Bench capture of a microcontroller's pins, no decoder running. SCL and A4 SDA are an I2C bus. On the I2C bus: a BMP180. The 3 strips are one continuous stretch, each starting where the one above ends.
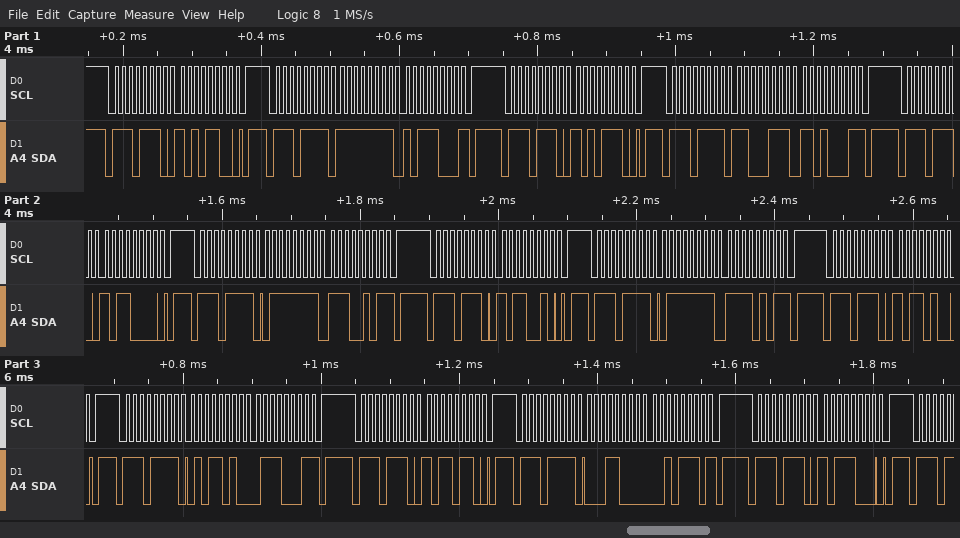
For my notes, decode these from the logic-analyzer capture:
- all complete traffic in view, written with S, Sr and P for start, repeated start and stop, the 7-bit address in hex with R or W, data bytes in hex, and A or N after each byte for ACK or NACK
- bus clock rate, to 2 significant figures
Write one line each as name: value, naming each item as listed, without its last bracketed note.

all complete traffic in view, written with S, Sr and P for start, repeated start and stop, the 7-bit address in hex with R or W, data bytes in hex, and A or N after each byte for ACK or NACK: S 77W A AC A P S 77R A FF A B8 N P S 77W A AE A P S 77R A C7 A D1 N P S 77W A B0 A P S 77R A 7F A E5 N P S 77W A B2 A P S 77R A 7F A F5 N P S 77W A B4 A P S 77R A 5A A 71 N P S 77W A B6 A P S 77R A 18 A 2E N P S 77W A B8 A P
bus clock rate, to 2 significant figures: 100 kHz
